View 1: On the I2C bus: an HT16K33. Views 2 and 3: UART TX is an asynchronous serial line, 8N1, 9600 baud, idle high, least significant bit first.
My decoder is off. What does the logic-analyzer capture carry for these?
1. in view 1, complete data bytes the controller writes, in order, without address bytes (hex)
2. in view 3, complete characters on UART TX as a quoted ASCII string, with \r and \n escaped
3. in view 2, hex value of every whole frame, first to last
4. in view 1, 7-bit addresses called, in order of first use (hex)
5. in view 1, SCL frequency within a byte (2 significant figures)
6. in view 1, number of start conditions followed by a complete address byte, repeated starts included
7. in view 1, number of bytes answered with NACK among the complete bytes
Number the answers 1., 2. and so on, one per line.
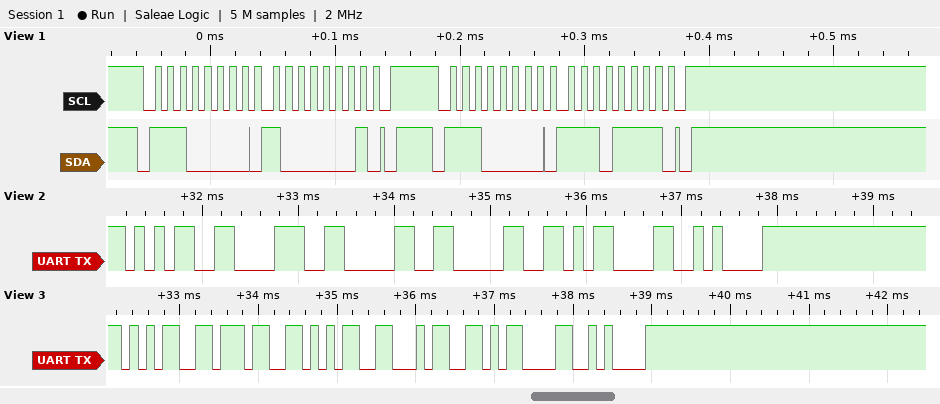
1. 81 EF
2. "5754\r\n"
3. 35 38 30 30 0D 0A
4. 0x70
5. 100 kHz
6. 2
7. 0
